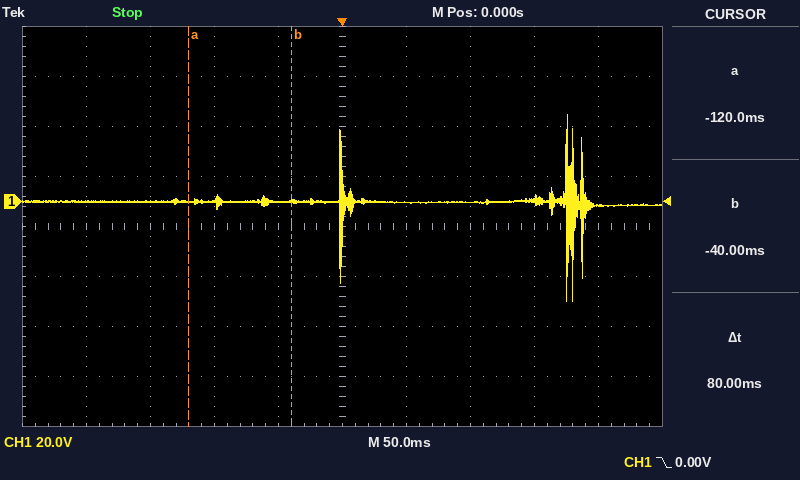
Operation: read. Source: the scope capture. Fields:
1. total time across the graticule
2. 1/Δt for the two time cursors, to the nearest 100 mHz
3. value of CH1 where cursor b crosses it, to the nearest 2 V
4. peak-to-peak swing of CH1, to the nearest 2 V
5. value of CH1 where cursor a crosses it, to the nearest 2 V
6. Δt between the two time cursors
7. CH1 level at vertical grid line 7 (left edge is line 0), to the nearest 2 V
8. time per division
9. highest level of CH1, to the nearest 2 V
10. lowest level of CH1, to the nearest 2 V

500 ms
12.5 Hz
0 V
74 V
0 V
80 ms
0 V
50 ms
34 V
-40 V
